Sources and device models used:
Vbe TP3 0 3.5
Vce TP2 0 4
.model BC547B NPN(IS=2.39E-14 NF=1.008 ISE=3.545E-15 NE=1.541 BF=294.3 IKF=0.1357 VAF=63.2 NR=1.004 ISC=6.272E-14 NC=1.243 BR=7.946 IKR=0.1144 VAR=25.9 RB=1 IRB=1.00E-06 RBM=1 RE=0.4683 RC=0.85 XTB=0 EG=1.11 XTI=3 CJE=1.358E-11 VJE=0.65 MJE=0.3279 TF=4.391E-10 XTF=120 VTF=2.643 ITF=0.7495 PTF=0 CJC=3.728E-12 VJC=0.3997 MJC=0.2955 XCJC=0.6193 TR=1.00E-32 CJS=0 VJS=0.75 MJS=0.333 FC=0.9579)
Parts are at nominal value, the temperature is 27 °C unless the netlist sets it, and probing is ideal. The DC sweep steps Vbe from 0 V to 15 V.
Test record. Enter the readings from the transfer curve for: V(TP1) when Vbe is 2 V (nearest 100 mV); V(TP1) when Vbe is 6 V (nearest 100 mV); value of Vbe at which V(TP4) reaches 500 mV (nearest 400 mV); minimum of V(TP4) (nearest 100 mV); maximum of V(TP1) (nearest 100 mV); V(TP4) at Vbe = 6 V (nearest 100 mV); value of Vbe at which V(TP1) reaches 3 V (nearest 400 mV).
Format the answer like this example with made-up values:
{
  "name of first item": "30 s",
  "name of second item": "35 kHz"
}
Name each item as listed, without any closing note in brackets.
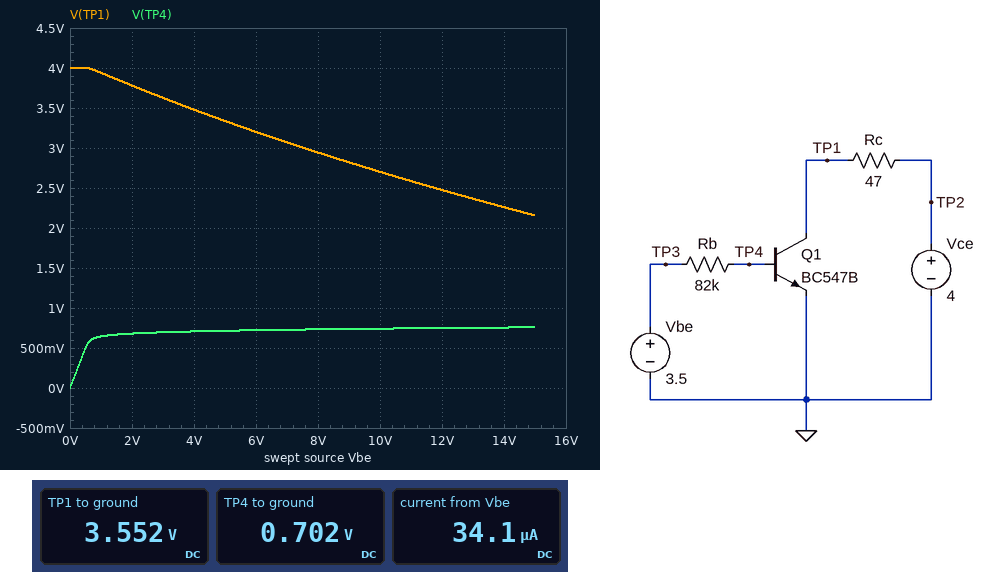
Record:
{
  "V(TP1) when Vbe is 2 V": "3.8 V",
  "V(TP1) when Vbe is 6 V": "3.2 V",
  "value of Vbe at which V(TP4) reaches 500 mV": "400 mV",
  "minimum of V(TP4)": "0 V",
  "maximum of V(TP1)": "4.0 V",
  "V(TP4) at Vbe = 6 V": "700 mV",
  "value of Vbe at which V(TP1) reaches 3 V": "7.6 V"
}
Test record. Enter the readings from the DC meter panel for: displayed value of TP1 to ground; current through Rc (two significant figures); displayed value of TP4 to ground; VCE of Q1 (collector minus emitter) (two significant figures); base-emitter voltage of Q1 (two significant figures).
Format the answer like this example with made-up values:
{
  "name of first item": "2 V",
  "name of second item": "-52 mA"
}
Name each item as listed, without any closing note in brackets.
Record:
{
  "displayed value of TP1 to ground": "3.552 V",
  "current through Rc": "9.5 mA",
  "displayed value of TP4 to ground": "0.702 V",
  "VCE of Q1 (collector minus emitter)": "3.6 V",
  "base-emitter voltage of Q1": "700 mV"
}
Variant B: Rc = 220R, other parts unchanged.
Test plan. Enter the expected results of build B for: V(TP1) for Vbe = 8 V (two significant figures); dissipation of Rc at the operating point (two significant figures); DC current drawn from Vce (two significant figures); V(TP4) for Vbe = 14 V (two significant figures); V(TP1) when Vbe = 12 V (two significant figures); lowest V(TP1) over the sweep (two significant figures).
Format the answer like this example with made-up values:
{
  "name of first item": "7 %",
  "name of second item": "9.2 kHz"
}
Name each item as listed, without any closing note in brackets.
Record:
{
  "V(TP1) for Vbe = 8 V": "160 mV",
  "dissipation of Rc at the operating point": "19 mW",
  "DC current drawn from Vce": "9.3 mA",
  "V(TP4) for Vbe = 14 V": "730 mV",
  "V(TP1) when Vbe = 12 V": "130 mV",
  "lowest V(TP1) over the sweep": "120 mV"
}
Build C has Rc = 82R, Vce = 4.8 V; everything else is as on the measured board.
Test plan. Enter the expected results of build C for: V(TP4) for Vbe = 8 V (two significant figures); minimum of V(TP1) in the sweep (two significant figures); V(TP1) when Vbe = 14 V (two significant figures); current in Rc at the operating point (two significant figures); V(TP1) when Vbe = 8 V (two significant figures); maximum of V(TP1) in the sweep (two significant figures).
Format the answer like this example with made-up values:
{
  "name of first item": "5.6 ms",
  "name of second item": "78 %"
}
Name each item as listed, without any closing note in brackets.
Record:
{
  "V(TP4) for Vbe = 8 V": "730 mV",
  "minimum of V(TP1) in the sweep": "1.6 V",
  "V(TP1) when Vbe = 14 V": "1.8 V",
  "current in Rc at the operating point": "9.6 mA",
  "V(TP1) when Vbe = 8 V": "3.0 V",
  "maximum of V(TP1) in the sweep": "4.8 V"
}
